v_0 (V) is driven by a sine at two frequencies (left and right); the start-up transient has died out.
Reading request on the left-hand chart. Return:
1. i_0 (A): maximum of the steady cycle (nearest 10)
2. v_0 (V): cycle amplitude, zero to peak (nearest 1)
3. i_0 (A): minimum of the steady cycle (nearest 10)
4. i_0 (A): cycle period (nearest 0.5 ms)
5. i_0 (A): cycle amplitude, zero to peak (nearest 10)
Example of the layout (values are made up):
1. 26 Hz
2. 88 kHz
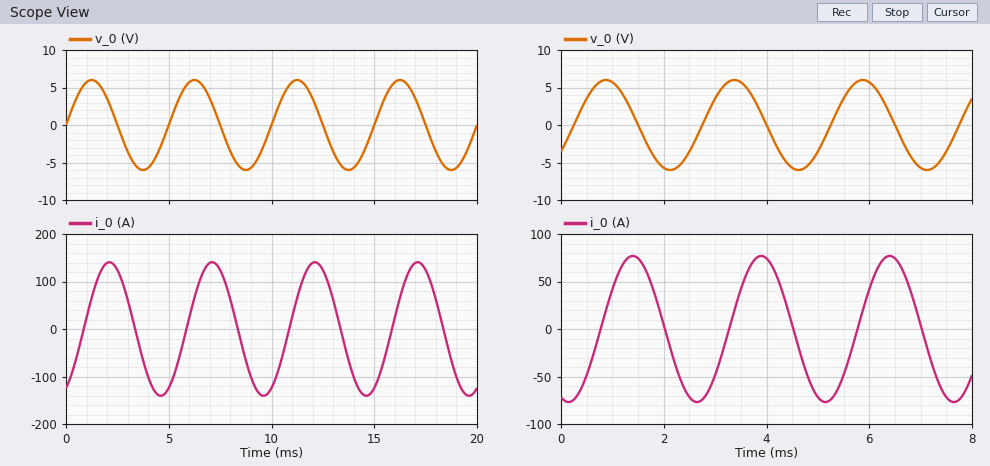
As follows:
1. 140
2. 6
3. -140
4. 5.0 ms
5. 140
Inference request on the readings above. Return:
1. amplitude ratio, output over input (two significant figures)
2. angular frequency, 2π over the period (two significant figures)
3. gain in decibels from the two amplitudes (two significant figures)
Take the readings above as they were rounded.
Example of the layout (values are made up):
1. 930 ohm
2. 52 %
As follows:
1. 23
2. 1.3 rad/ms
3. 27 dB
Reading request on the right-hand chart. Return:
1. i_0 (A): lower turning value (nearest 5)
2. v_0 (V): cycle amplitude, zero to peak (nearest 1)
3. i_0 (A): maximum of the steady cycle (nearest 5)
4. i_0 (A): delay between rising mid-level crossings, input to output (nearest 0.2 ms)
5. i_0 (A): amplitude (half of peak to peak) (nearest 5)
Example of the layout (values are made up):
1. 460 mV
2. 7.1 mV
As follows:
1. -75
2. 6
3. 75
4. 0.6 ms
5. 75
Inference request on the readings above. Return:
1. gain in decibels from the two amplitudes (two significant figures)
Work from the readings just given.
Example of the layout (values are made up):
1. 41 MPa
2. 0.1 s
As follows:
1. 22 dB
